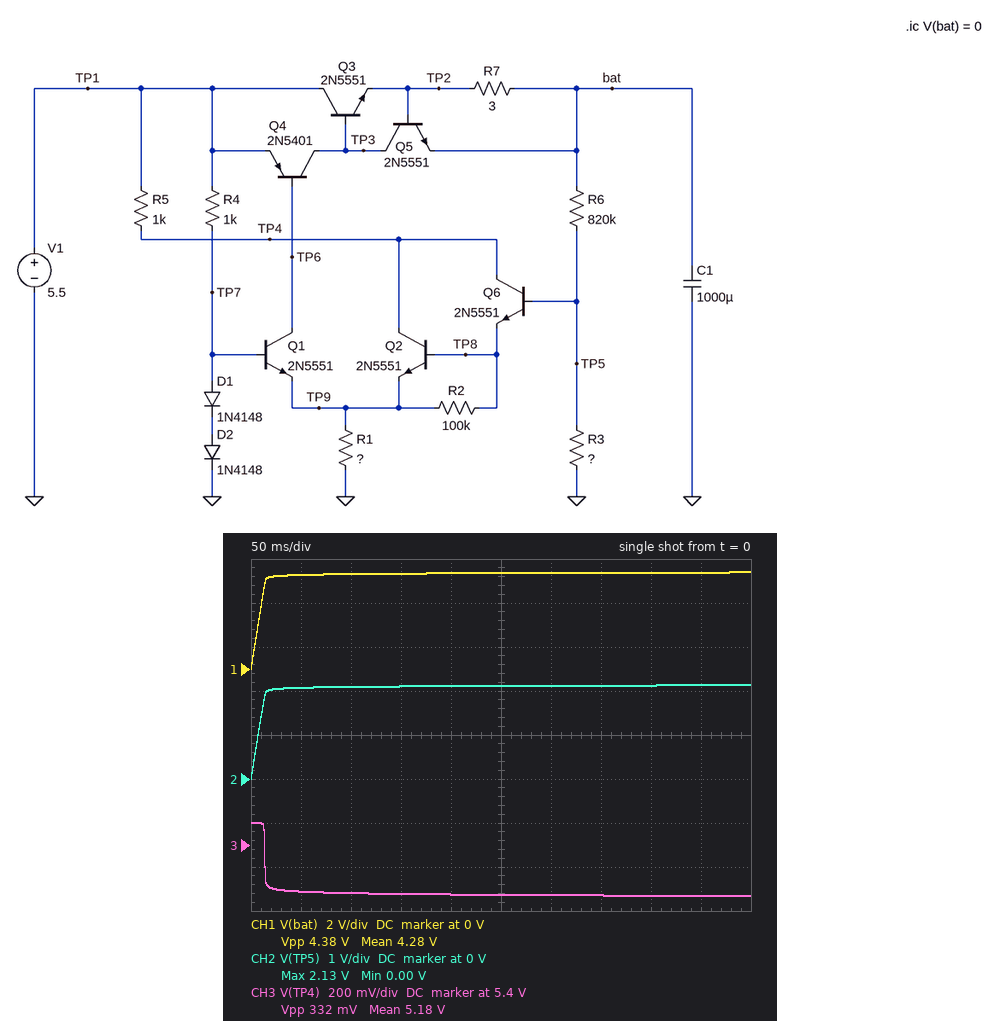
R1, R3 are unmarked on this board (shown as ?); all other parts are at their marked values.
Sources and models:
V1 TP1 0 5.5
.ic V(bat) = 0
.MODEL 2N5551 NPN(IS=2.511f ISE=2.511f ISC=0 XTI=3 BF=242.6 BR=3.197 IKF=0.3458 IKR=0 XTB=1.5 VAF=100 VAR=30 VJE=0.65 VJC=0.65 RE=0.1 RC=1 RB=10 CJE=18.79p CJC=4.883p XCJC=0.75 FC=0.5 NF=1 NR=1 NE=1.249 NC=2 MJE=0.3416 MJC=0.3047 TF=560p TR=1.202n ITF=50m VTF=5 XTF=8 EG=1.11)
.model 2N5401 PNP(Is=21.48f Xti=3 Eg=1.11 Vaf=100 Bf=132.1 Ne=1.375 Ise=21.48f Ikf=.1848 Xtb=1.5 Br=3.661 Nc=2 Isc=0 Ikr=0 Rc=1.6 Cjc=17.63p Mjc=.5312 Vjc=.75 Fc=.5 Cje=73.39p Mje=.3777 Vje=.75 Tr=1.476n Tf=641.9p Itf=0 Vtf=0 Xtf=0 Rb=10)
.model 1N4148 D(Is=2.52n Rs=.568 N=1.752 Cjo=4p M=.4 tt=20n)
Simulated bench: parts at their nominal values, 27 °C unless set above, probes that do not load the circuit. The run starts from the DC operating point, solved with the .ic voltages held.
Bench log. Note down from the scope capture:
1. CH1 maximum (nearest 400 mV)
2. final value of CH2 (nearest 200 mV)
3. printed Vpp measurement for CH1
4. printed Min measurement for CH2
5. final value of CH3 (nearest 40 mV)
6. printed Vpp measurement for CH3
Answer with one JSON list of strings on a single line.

["4.4 V", "2.2 V", "4.38 V", "0.00 V", "5.16 V", "332 mV"]
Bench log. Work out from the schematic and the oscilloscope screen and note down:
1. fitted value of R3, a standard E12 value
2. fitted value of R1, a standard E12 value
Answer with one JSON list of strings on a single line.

["820 kΩ", "2.7 kΩ"]
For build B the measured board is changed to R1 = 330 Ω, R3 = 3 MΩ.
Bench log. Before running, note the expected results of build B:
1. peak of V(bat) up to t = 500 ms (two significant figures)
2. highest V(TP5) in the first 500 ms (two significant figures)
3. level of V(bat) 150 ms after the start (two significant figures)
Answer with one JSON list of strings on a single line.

["3.2 V", "2.2 V", "3.1 V"]
